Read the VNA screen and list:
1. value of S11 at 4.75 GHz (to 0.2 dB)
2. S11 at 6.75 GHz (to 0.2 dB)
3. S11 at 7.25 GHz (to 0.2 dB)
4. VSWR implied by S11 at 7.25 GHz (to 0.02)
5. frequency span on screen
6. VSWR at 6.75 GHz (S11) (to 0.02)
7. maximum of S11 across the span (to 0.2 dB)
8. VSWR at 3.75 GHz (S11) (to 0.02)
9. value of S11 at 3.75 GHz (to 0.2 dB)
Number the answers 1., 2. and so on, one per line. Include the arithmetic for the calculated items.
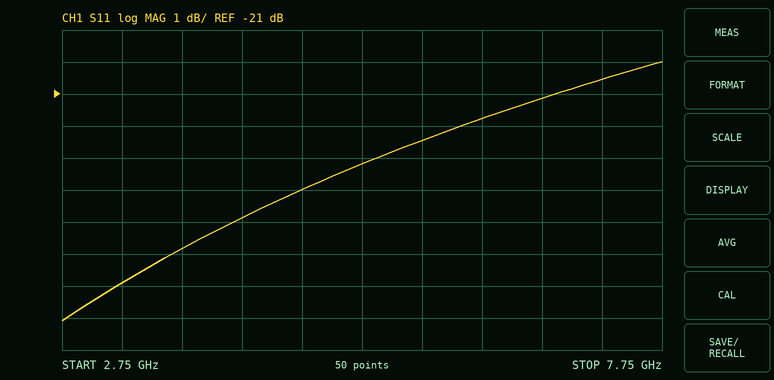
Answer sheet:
1. -24.0 dB
2. -21.2 dB
3. -20.6 dB
4. |Γ| = 10^(-20.6/20) = 0.0933; VSWR = (1 + 0.0933)/(1 − 0.0933) ≈ 1.21, so 1.20 to the nearest 0.02
5. 5 GHz
6. |Γ| = 10^(-21.2/20) = 0.0871; VSWR = (1 + 0.0871)/(1 − 0.0871) ≈ 1.19, so 1.20 to the nearest 0.02
7. -20.0 dB
8. |Γ| = 10^(-25.8/20) = 0.0513; VSWR = (1 + 0.0513)/(1 − 0.0513) ≈ 1.11, so 1.10 to the nearest 0.02
9. -25.8 dB
